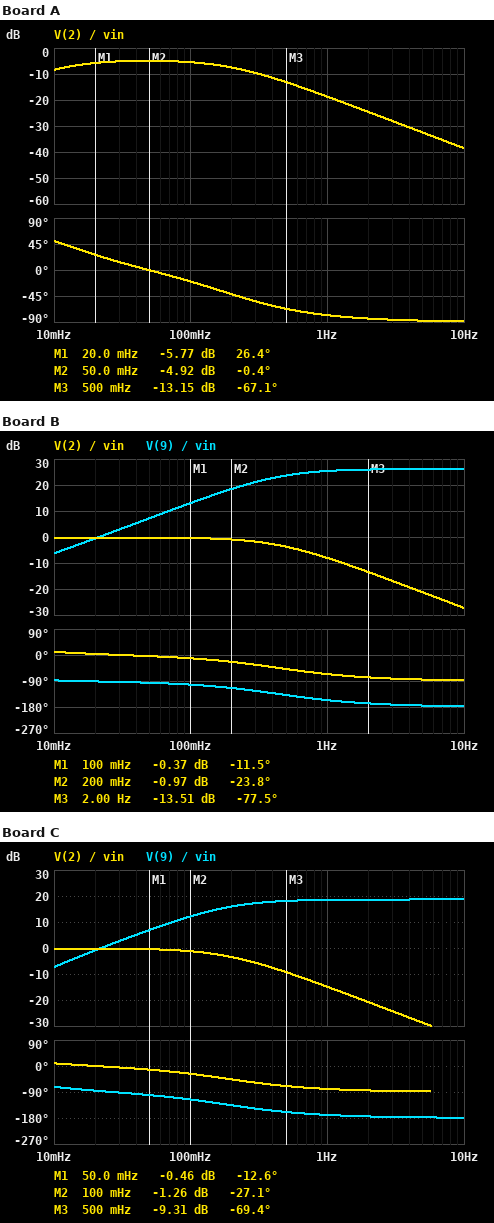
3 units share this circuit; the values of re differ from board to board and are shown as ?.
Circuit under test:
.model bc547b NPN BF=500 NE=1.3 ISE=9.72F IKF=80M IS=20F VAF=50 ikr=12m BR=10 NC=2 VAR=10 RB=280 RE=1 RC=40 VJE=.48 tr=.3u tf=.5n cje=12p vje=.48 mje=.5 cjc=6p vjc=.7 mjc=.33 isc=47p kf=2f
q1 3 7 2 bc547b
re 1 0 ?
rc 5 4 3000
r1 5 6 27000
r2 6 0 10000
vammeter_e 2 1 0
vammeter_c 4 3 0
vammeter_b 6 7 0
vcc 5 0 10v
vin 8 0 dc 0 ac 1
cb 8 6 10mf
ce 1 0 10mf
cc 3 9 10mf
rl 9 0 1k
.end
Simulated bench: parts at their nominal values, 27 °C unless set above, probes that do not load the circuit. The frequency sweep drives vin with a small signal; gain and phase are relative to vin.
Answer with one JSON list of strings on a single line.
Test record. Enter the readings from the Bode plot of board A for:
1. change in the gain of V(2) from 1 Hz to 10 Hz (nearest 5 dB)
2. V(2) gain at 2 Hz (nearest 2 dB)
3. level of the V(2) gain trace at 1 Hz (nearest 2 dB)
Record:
["-20 dB", "-24 dB", "-18 dB"]
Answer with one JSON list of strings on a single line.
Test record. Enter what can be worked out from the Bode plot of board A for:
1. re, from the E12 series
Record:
["680 Ω"]
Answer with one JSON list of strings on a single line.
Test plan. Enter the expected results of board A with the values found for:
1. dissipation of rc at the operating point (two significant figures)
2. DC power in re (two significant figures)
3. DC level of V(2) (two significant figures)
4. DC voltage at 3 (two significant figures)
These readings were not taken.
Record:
["21 mW", "4.9 mW", "1.8 V", "2.0 V"]
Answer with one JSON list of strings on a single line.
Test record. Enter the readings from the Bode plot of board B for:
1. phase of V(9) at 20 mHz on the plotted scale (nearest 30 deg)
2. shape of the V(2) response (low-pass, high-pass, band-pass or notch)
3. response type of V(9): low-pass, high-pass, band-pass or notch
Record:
["-90 deg", "low-pass", "high-pass"]
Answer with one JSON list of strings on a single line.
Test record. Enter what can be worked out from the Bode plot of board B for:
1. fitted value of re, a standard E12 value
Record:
["2.7 kΩ"]
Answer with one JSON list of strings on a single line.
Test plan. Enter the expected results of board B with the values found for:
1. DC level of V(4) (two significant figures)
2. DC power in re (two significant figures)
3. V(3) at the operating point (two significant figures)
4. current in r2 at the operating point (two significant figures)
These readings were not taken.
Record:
["7.7 V", "1.6 mW", "7.7 V", "270 µA"]
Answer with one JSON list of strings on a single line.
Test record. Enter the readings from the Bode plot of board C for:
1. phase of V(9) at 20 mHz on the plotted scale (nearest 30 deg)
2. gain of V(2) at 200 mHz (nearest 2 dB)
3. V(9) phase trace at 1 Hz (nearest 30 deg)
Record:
["-90 deg", "-4 dB", "-180 deg"]
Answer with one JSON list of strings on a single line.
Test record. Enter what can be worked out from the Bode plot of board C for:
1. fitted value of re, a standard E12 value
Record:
["6.8 kΩ"]
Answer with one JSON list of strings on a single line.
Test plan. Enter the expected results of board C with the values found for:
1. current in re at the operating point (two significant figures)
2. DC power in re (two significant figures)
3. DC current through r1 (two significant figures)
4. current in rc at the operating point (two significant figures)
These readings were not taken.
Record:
["310 µA", "640 µW", "270 µA", "310 µA"]
